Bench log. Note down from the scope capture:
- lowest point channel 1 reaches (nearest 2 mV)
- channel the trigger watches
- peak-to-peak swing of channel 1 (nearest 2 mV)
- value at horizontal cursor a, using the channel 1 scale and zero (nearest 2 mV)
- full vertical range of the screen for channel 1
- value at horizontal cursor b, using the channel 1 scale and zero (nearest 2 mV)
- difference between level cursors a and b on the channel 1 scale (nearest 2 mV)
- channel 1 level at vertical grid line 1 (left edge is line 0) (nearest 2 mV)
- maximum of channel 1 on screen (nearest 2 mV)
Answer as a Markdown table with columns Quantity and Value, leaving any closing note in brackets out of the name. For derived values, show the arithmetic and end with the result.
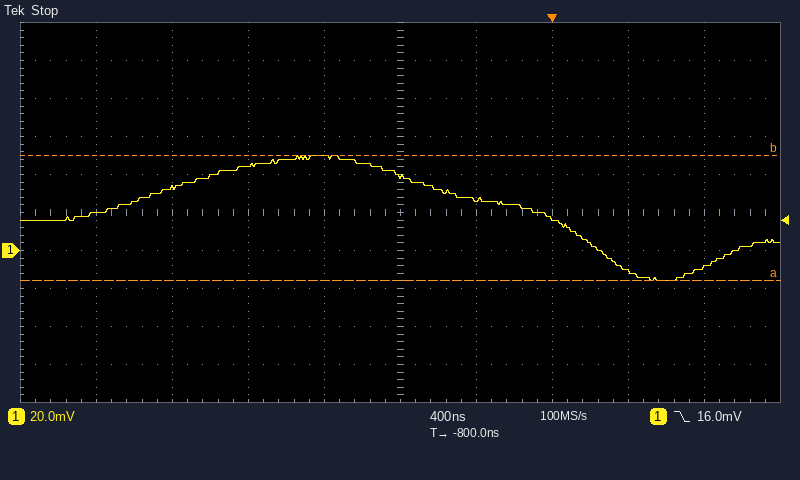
| Quantity | Value |
|---|---|
| lowest point channel 1 reaches | -16 mV |
| channel the trigger watches | channel 1 |
| peak-to-peak swing of channel 1 | 50 mV − (-16 mV) = 66 mV |
| value at horizontal cursor a, using the channel 1 scale and zero | -16 mV |
| full vertical range of the screen for channel 1 | 200 mV |
| value at horizontal cursor b, using the channel 1 scale and zero | 50 mV |
| difference between level cursors a and b on the channel 1 scale | 66 mV |
| channel 1 level at vertical grid line 1 (left edge is line 0) | 20 mV |
| maximum of channel 1 on screen | 50 mV |
